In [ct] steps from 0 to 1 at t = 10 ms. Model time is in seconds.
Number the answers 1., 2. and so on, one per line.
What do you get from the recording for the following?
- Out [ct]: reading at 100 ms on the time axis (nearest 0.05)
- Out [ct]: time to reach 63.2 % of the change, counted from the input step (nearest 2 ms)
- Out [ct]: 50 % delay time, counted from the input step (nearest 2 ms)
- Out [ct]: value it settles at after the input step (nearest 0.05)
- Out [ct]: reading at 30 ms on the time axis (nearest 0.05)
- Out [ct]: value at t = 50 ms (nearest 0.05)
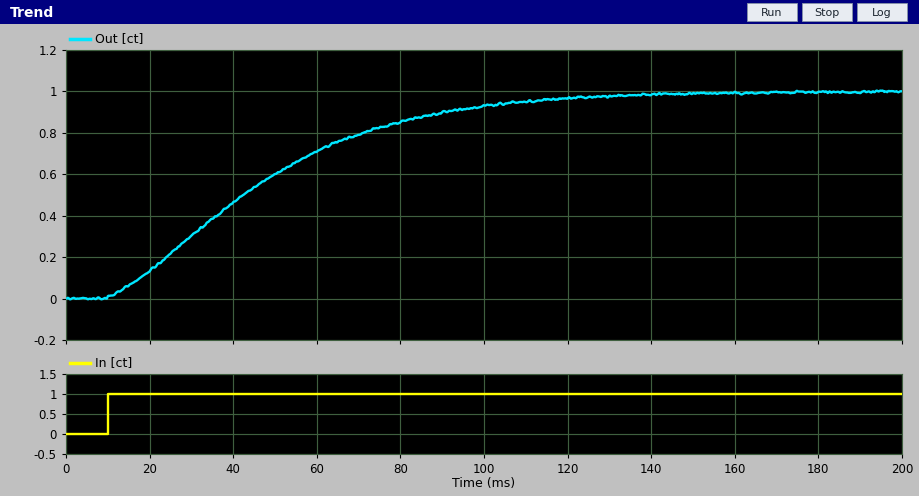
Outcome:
1. 0.95
2. 42 ms
3. 32 ms
4. 1.00
5. 0.30
6. 0.60
